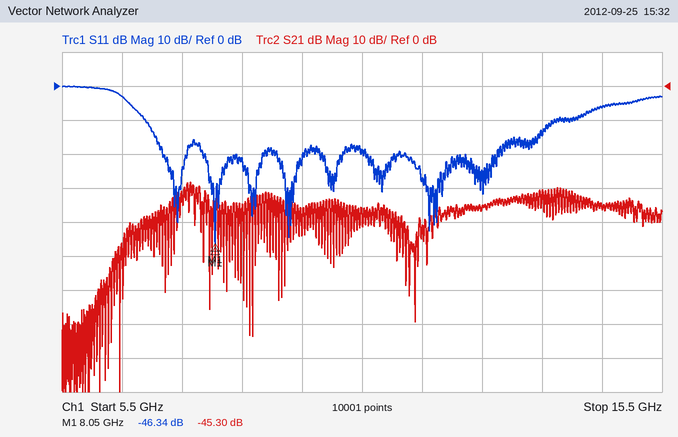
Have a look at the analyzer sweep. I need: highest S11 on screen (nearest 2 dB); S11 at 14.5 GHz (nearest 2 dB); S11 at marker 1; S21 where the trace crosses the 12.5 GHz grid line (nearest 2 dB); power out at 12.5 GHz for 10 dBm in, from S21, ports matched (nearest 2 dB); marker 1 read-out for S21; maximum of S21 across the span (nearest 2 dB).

0 dB
-6 dB
-46.34 dB
-36 dB
-26 dBm
-45.30 dB
-28 dB
